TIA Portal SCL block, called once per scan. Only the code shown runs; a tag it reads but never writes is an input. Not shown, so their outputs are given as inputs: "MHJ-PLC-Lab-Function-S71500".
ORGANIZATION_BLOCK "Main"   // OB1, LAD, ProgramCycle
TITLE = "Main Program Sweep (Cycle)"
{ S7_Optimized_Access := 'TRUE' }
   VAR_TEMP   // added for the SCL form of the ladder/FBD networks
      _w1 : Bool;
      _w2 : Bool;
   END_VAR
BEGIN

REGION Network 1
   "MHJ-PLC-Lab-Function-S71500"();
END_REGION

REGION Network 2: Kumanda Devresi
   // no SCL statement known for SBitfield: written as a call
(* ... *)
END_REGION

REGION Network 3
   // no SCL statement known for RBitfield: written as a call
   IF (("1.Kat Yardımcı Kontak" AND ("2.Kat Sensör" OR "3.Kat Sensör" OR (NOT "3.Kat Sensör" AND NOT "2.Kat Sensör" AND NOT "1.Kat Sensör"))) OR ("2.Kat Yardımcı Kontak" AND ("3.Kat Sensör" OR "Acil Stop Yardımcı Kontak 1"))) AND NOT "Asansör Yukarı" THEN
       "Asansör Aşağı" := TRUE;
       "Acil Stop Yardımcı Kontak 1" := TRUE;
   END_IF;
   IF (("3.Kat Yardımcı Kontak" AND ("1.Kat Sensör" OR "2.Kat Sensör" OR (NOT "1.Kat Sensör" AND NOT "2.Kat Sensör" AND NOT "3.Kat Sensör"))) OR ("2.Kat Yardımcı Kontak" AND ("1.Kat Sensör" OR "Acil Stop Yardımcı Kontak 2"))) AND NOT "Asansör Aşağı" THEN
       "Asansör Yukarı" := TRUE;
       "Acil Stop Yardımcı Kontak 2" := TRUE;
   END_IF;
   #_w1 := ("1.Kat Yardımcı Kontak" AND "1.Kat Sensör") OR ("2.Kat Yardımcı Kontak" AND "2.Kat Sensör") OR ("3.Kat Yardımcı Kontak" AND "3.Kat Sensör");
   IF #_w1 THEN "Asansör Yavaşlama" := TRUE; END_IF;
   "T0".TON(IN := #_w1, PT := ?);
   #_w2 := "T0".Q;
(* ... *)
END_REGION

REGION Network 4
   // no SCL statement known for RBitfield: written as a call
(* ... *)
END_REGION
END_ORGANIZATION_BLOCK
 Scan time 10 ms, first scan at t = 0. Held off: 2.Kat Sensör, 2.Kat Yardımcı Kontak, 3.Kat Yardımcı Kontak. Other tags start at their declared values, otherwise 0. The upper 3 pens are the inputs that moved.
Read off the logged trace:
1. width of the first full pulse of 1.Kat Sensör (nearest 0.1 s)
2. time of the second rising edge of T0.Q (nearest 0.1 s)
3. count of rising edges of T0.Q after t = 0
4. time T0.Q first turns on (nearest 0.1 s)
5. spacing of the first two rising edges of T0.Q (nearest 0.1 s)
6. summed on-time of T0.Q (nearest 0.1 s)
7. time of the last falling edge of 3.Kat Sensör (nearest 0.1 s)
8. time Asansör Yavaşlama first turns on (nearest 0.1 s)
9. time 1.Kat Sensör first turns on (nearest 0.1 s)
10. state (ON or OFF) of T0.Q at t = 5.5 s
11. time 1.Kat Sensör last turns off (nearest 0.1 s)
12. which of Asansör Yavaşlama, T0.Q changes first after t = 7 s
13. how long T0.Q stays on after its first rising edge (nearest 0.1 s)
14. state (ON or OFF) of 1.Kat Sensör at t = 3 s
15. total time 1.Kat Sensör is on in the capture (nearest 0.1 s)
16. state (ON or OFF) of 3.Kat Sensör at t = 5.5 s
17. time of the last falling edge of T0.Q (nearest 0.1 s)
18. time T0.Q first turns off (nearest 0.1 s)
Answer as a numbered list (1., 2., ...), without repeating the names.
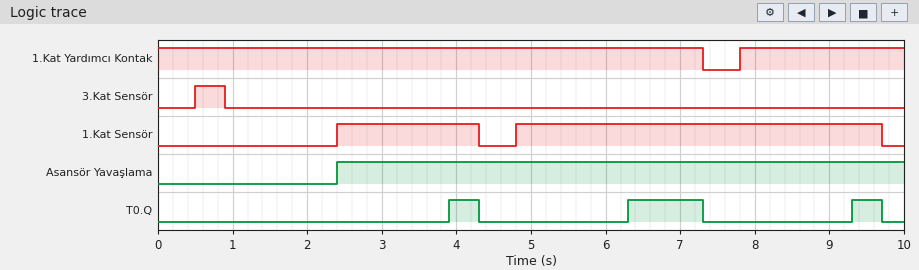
1. 1.9 s
2. 6.3 s
3. 3
4. 3.9 s
5. 2.4 s
6. 1.8 s
7. 0.9 s
8. 2.4 s
9. 2.4 s
10. OFF
11. 9.7 s
12. T0.Q
13. 0.4 s
14. ON
15. 6.8 s
16. OFF
17. 9.7 s
18. 4.3 s
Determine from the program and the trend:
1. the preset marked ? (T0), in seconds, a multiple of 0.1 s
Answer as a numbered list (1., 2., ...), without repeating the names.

1. 1.5 s
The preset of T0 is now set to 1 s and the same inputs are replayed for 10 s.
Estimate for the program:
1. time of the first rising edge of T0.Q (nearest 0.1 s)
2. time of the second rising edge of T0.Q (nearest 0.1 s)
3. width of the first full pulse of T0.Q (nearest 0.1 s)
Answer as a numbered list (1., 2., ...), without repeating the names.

1. 3.4 s
2. 5.8 s
3. 0.9 s
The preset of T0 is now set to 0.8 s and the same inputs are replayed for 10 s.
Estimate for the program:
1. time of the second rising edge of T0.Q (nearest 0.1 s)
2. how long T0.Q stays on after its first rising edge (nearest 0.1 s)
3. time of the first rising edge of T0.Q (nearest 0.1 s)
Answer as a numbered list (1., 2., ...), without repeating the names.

1. 5.6 s
2. 1.1 s
3. 3.2 s
